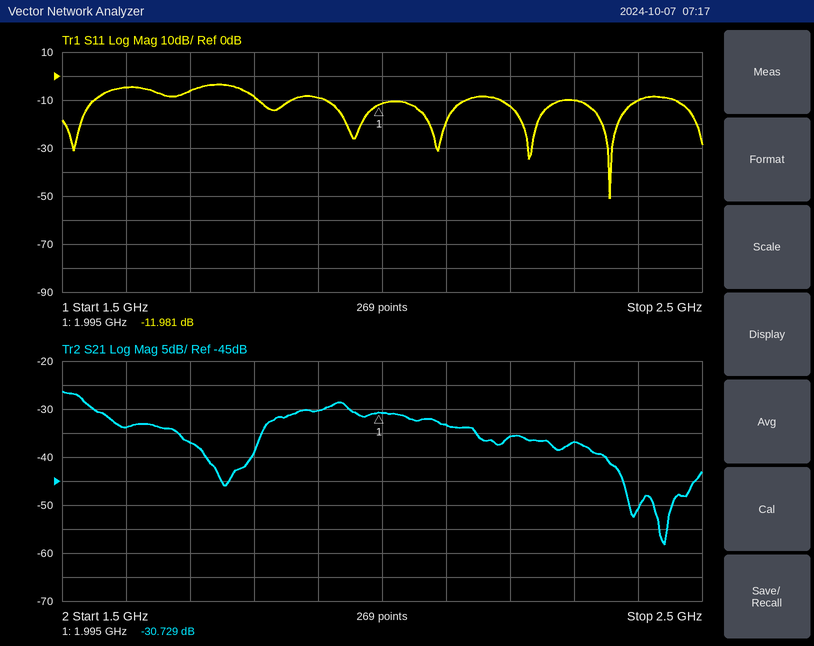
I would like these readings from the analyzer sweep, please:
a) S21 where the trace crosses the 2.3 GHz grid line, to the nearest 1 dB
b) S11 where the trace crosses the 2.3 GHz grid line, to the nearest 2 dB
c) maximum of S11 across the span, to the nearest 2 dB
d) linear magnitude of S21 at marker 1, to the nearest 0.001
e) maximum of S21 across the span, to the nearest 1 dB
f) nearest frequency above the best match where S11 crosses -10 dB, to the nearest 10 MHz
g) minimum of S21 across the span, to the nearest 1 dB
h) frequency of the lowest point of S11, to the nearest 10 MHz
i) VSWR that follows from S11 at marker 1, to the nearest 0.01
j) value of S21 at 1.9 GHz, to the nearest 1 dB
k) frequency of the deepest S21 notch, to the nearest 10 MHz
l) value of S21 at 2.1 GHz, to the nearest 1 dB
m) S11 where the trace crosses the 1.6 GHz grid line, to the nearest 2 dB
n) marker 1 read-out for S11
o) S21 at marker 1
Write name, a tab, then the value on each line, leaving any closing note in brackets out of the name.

S21 where the trace crosses the 2.3 GHz grid line, to the nearest 1 dB	-37 dB
S11 where the trace crosses the 2.3 GHz grid line, to the nearest 2 dB	-10 dB
maximum of S11 across the span, to the nearest 2 dB	-4 dB
linear magnitude of S21 at marker 1, to the nearest 0.001	0.029
maximum of S21 across the span, to the nearest 1 dB	-26 dB
nearest frequency above the best match where S11 crosses -10 dB, to the nearest 10 MHz	2.40 GHz
minimum of S21 across the span, to the nearest 1 dB	-58 dB
frequency of the lowest point of S11, to the nearest 10 MHz	2.36 GHz
VSWR that follows from S11 at marker 1, to the nearest 0.01	1.67
value of S21 at 1.9 GHz, to the nearest 1 dB	-30 dB
frequency of the deepest S21 notch, to the nearest 10 MHz	2.44 GHz
value of S21 at 2.1 GHz, to the nearest 1 dB	-33 dB
S11 where the trace crosses the 1.6 GHz grid line, to the nearest 2 dB	-4 dB
marker 1 read-out for S11	-11.981 dB
S21 at marker 1	-30.729 dB
